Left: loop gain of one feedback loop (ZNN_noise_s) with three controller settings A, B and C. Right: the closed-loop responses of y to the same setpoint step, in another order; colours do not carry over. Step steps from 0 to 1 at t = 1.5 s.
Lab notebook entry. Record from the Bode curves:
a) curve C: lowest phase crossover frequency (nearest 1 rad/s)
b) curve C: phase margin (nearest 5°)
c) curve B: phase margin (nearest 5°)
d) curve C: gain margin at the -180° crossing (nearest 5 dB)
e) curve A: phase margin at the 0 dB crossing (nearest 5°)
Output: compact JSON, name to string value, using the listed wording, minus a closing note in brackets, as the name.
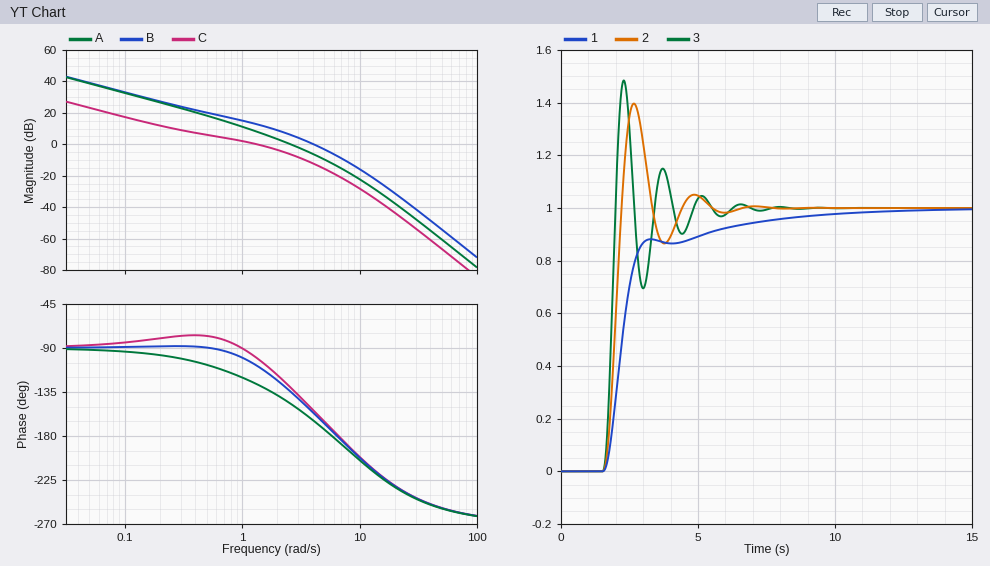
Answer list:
{"curve C: lowest phase crossover frequency": "7 rad/s", "curve C: phase margin": "80°", "curve B: phase margin": "25°", "curve C: gain margin at the -180° crossing": "20 dB", "curve A: phase margin at the 0 dB crossing": "35°"}
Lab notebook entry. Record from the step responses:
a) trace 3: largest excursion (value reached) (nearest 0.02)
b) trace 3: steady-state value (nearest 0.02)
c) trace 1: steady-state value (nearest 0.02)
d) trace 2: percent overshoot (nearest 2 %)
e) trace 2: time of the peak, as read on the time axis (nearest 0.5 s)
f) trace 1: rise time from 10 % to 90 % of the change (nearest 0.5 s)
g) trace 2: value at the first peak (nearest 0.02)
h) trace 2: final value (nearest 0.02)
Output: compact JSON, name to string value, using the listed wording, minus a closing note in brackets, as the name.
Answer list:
{"trace 3: largest excursion (value reached)": "1.48", "trace 3: steady-state value": "1.00", "trace 1: steady-state value": "1.00", "trace 2: percent overshoot": "40 %", "trace 2: time of the peak, as read on the time axis": "2.5 s", "trace 1: rise time from 10 % to 90 % of the change": "3.5 s", "trace 2: value at the first peak": "1.40", "trace 2: final value": "1.00"}
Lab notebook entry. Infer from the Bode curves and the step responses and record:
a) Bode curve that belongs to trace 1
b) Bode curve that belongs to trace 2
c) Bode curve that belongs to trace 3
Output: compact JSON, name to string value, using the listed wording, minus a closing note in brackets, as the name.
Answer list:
{"Bode curve that belongs to trace 1": "C", "Bode curve that belongs to trace 2": "A", "Bode curve that belongs to trace 3": "B"}
